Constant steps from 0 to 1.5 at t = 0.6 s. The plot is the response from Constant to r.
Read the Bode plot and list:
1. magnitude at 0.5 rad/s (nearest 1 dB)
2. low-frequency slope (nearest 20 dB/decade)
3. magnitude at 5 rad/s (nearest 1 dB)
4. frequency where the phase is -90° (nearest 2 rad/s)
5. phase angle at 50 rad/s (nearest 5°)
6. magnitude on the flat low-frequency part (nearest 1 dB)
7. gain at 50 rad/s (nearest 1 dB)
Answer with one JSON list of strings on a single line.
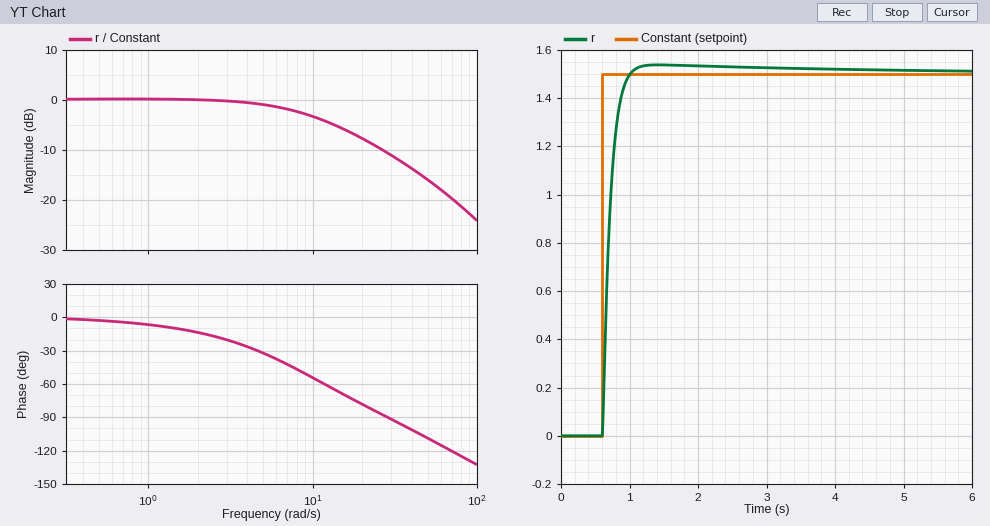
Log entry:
["0 dB", "0 dB/decade", "-1 dB", "28 rad/s", "-110°", "0 dB", "-16 dB"]
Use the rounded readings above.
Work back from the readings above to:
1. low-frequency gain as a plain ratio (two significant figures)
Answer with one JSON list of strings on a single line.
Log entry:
["1.0"]
